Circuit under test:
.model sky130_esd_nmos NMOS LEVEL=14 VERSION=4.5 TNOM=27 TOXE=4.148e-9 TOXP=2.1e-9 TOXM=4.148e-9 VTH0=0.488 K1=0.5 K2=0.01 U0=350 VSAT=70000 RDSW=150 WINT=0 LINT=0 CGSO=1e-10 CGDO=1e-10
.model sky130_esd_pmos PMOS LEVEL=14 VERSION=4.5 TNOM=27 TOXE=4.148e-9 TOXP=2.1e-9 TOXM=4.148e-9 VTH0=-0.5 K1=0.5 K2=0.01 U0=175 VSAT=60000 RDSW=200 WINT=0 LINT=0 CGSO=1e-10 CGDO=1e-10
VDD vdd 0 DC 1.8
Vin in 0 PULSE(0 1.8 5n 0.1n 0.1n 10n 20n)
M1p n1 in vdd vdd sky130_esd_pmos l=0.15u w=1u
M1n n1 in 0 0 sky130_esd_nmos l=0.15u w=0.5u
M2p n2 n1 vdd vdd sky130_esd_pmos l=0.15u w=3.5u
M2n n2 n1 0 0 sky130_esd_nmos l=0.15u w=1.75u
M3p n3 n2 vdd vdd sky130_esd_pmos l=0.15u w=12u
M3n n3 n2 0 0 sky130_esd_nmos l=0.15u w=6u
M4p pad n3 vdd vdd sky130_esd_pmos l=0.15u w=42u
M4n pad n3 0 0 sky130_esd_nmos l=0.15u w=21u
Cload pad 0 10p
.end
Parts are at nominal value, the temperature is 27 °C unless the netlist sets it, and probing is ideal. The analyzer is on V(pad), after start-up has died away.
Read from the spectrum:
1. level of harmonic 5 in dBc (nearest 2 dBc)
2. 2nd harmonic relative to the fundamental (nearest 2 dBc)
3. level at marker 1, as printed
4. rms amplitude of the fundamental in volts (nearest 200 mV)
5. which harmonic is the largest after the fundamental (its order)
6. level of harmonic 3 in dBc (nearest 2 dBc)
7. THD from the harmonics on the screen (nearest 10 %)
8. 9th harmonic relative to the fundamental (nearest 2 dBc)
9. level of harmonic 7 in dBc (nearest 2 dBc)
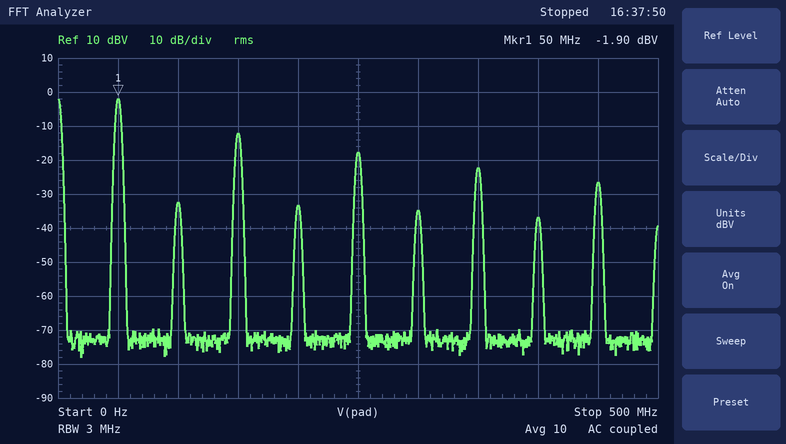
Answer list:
-16 dBc
-30 dBc
-1.90 dBV
800 mV
3
-10 dBc
40 %
-24 dBc
-20 dBc
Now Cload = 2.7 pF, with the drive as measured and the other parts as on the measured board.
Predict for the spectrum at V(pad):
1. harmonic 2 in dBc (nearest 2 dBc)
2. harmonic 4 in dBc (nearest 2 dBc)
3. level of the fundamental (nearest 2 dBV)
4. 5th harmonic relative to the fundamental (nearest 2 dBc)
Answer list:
-34 dBc
-34 dBc
-2 dBV
-14 dBc
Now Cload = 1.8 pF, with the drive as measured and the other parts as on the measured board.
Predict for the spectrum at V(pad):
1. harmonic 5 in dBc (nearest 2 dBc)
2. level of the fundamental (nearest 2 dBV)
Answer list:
-14 dBc
-2 dBV
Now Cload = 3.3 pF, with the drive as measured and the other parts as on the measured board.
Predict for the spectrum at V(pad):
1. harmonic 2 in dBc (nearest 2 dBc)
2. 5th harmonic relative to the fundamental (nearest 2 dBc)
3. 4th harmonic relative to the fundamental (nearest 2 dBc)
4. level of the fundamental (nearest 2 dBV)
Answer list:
-34 dBc
-14 dBc
-34 dBc
-2 dBV
